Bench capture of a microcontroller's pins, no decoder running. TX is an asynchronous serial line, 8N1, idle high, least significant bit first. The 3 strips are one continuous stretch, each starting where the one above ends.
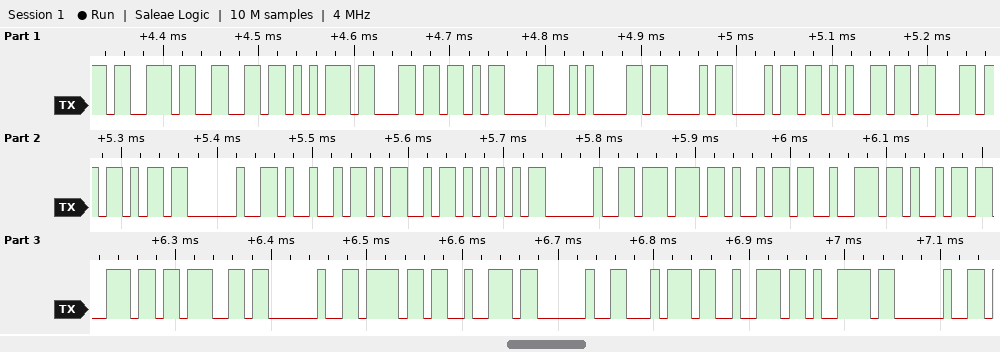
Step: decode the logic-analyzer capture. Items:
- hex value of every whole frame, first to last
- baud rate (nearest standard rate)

73 66 75 6C 0D 0A 43 68 65 63 6B 20 49 4D 55 20 77 69 72 69 6E 67 20 6F 72 20 74 72 79 20
115200 baud
